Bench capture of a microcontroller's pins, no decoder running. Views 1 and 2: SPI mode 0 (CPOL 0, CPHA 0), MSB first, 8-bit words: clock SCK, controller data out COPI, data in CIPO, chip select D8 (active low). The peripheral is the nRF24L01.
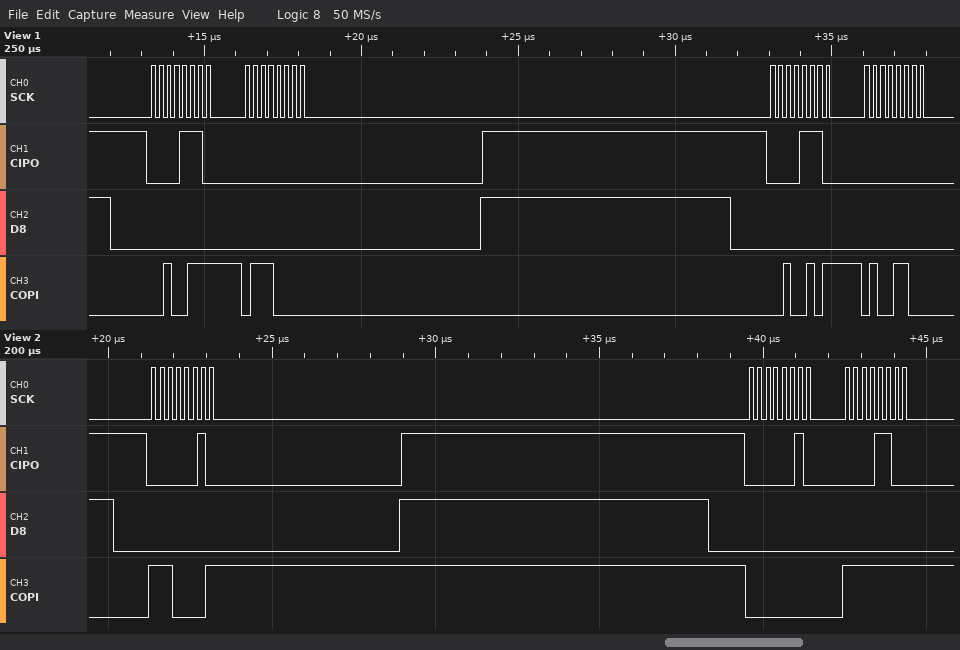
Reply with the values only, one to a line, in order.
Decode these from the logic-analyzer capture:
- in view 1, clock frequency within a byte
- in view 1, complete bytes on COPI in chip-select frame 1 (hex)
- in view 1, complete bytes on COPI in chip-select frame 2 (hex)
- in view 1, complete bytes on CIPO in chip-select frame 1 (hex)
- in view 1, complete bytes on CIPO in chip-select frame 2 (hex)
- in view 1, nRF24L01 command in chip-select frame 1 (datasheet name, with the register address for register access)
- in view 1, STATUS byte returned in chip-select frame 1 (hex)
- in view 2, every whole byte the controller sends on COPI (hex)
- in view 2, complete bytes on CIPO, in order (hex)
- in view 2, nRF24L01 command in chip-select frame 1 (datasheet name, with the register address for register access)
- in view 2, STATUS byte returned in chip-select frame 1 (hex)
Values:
4 MHz
27 70
25 4C
0E 00
0E 00
W_REGISTER 0x07
0x0E
E1 00 FF
02 02 0C
FLUSH_TX
0x02
